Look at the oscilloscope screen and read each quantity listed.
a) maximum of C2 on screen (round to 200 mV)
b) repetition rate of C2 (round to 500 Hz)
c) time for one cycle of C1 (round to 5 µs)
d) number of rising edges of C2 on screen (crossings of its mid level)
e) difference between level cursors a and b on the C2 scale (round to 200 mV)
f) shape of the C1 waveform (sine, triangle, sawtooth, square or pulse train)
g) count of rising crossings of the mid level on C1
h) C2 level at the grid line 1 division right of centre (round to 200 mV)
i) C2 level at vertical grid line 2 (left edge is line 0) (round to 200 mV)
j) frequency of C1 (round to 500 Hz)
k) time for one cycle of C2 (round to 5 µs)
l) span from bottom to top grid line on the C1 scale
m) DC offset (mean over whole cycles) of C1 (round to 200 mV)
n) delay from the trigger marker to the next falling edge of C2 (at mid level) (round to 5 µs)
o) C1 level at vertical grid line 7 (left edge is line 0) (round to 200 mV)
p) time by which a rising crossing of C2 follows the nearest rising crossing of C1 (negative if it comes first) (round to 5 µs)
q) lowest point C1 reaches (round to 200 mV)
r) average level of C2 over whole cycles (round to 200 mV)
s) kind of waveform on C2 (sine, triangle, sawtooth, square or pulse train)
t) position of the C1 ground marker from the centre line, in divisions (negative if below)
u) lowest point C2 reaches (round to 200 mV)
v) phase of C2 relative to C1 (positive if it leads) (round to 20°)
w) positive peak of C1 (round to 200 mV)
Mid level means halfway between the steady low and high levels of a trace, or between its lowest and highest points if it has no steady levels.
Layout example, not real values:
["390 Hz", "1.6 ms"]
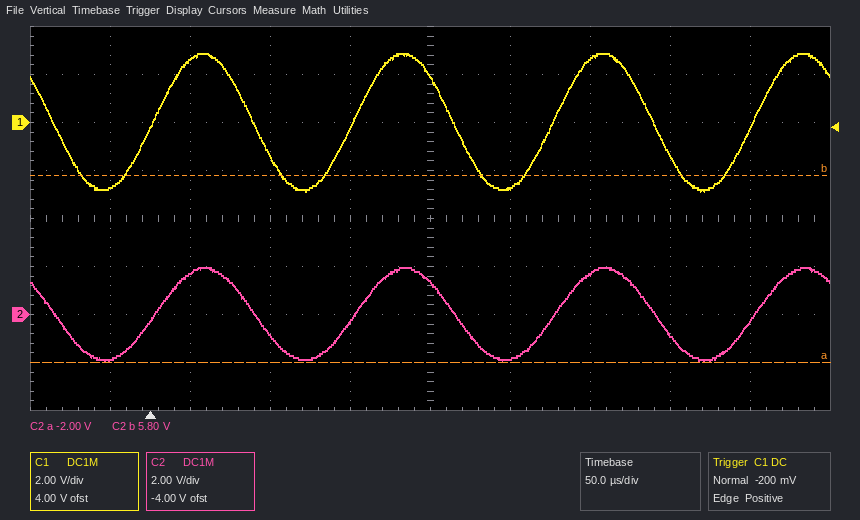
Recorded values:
["2.0 V", "8.0 kHz", "125 µs", "4", "7.8 V", "sine", "4", "-1.8 V", "1.8 V", "8.0 kHz", "125 µs", "16 V", "0.0 V", "65 µs", "2.6 V", "0 µs", "-2.8 V", "0.0 V", "sine", "+2.0 div", "-2.0 V", "0°", "2.8 V"]
